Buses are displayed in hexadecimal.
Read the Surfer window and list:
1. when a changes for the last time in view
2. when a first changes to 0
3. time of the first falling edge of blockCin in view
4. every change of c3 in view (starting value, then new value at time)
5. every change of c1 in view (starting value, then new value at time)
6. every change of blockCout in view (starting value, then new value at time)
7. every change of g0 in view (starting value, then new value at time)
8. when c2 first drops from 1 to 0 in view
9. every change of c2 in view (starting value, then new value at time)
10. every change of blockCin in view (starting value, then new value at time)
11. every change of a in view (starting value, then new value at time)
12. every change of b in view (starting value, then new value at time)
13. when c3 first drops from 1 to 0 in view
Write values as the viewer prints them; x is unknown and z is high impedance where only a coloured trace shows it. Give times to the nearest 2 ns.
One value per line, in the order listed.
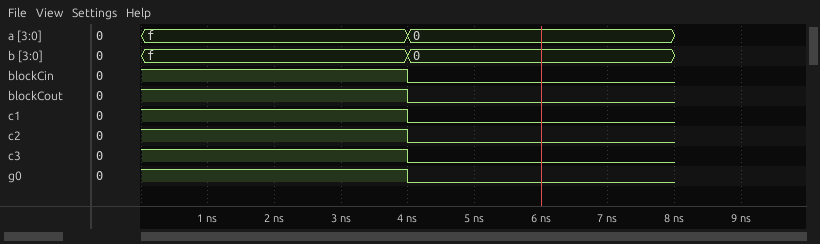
4 ns
4 ns
4 ns
1, 0 at 4 ns
1, 0 at 4 ns
1, 0 at 4 ns
1, 0 at 4 ns
4 ns
1, 0 at 4 ns
1, 0 at 4 ns
f, 0 at 4 ns
f, 0 at 4 ns
4 ns
